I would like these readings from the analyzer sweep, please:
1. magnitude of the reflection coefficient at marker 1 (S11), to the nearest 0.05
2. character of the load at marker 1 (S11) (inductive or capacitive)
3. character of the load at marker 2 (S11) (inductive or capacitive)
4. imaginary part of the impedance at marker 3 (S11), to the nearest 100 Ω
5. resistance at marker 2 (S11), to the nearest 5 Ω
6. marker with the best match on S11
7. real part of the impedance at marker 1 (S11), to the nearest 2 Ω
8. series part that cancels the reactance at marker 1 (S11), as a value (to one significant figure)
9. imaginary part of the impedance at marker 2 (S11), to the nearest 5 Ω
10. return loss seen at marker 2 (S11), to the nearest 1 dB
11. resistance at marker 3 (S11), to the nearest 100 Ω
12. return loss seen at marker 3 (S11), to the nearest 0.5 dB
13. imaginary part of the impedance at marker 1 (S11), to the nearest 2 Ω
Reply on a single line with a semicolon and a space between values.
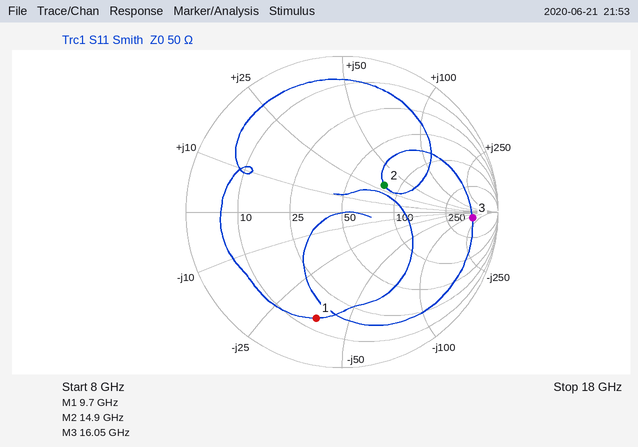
0.70; capacitive; inductive; -100 Ω; 80 Ω; marker 2; 14 Ω; 600 pH; +30 Ω; 10 dB; 500 Ω; 1.5 dB; -38 Ω
